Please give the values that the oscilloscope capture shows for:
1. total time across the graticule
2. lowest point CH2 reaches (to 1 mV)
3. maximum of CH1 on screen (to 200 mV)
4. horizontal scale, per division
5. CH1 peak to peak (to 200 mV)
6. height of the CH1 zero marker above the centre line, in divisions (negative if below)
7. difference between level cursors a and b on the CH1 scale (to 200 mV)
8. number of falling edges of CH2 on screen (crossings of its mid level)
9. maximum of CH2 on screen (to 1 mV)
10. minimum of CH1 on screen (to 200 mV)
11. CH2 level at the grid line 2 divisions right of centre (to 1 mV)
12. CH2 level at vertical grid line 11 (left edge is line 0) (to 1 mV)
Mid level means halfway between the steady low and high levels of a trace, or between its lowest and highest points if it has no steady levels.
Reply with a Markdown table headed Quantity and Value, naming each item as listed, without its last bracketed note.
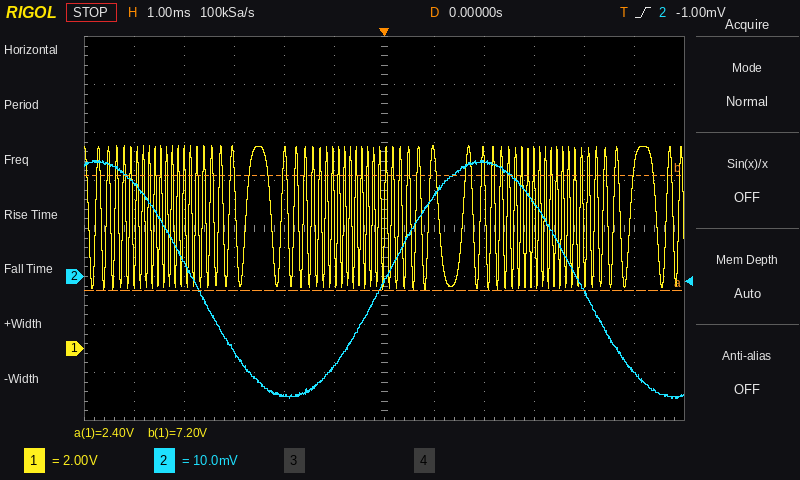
| Quantity | Value |
|---|---|
| total time across the graticule | 12 ms |
| lowest point CH2 reaches | -25 mV |
| maximum of CH1 on screen | 8.4 V |
| horizontal scale, per division | 1 ms |
| CH1 peak to peak | 6.0 V |
| height of the CH1 zero marker above the centre line, in divisions | -2.5 div |
| difference between level cursors a and b on the CH1 scale | 4.8 V |
| number of falling edges of CH2 on screen | 2 |
| maximum of CH2 on screen | 24 mV |
| minimum of CH1 on screen | 2.4 V |
| CH2 level at the grid line 2 divisions right of centre | 24 mV |
| CH2 level at vertical grid line 11 (left edge is line 0) | -20 mV |
